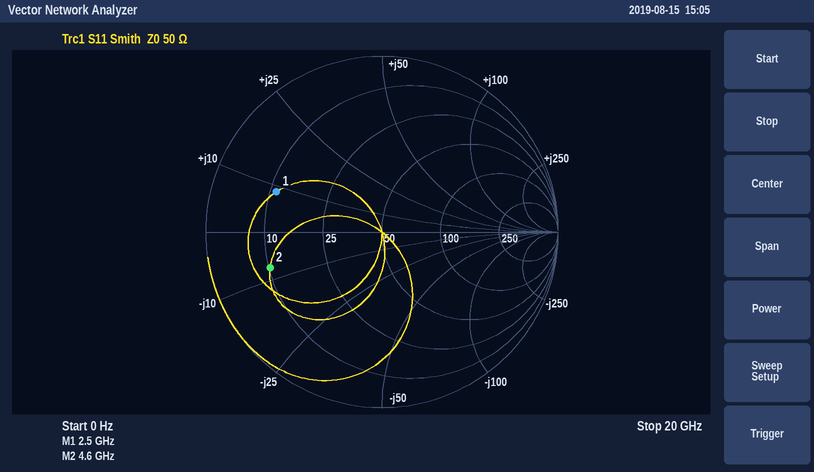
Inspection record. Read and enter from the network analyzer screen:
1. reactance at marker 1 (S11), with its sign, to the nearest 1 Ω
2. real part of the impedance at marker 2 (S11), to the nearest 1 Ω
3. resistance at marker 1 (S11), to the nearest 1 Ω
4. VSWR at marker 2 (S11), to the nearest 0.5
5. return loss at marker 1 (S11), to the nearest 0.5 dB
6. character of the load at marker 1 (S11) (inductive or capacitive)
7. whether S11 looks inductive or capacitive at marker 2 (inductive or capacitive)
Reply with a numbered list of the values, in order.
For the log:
1. +9 Ω
2. 10 Ω
3. 11 Ω
4. 5.0
5. 4.0 dB
6. inductive
7. capacitive
